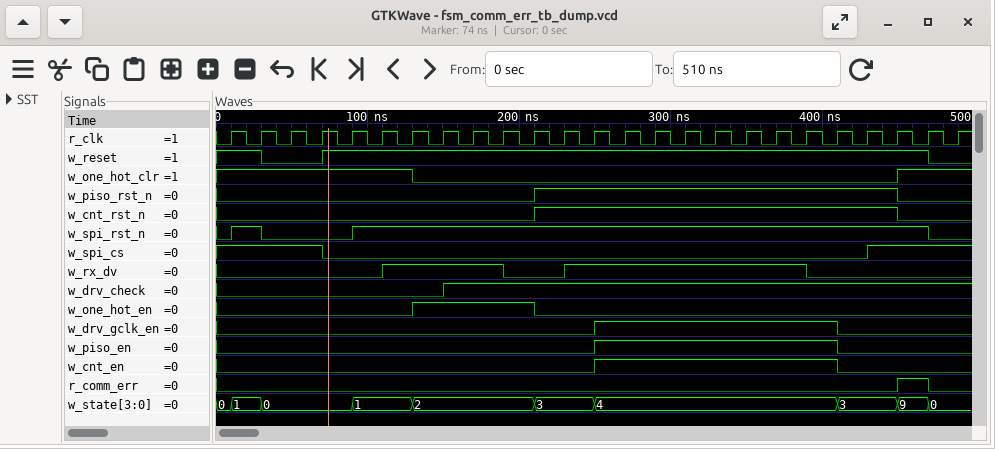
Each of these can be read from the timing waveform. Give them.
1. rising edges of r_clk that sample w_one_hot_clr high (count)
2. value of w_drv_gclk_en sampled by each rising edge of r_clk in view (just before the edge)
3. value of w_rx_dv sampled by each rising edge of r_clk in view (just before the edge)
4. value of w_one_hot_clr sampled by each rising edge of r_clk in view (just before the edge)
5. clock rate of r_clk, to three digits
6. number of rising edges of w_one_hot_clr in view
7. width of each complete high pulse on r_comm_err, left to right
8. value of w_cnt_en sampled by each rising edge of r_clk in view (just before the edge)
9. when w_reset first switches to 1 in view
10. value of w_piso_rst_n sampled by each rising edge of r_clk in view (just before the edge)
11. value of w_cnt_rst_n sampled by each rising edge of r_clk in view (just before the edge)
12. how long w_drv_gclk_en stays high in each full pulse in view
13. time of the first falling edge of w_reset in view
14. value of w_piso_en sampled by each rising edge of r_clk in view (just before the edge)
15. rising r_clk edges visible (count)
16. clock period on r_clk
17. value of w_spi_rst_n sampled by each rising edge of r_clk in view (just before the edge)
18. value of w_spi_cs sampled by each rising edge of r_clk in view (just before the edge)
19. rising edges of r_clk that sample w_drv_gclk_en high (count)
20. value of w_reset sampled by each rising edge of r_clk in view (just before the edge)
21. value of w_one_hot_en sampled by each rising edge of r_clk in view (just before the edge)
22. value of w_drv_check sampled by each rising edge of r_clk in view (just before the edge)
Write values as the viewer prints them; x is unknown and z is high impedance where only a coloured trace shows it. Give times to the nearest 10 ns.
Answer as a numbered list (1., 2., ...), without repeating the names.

1. 9
2. 0 0 0 0 0 0 0 0 0 0 0 0 0 1 1 1 1 1 1 1 1 0 0 0 0
3. 0 0 0 0 0 0 1 1 1 1 0 0 1 1 1 1 1 1 1 1 0 0 0 0 0
4. 1 1 1 1 1 1 1 0 0 0 0 0 0 0 0 0 0 0 0 0 0 0 0 1 1
5. 50.0 MHz
6. 1
7. 20 ns
8. 0 0 0 0 0 0 0 0 0 0 0 0 0 1 1 1 1 1 1 1 1 0 0 0 0
9. 70 ns
10. 0 0 0 0 0 0 0 0 0 0 0 1 1 1 1 1 1 1 1 1 1 1 1 0 0
11. 0 0 0 0 0 0 0 0 0 0 0 1 1 1 1 1 1 1 1 1 1 1 1 0 0
12. 160 ns
13. 30 ns
14. 0 0 0 0 0 0 0 0 0 0 0 0 0 1 1 1 1 1 1 1 1 0 0 0 0
15. 25
16. 20 ns
17. 0 1 0 0 0 1 1 1 1 1 1 1 1 1 1 1 1 1 1 1 1 1 1 1 0
18. 1 1 1 1 0 0 0 0 0 0 0 0 0 0 0 0 0 0 0 0 0 0 1 1 1
19. 8
20. 1 1 0 0 1 1 1 1 1 1 1 1 1 1 1 1 1 1 1 1 1 1 1 1 0
21. 0 0 0 0 0 0 0 1 1 1 1 0 0 0 0 0 0 0 0 0 0 0 0 0 0
22. 0 0 0 0 0 0 0 0 1 1 1 1 1 1 1 1 1 1 1 1 1 1 1 1 1
